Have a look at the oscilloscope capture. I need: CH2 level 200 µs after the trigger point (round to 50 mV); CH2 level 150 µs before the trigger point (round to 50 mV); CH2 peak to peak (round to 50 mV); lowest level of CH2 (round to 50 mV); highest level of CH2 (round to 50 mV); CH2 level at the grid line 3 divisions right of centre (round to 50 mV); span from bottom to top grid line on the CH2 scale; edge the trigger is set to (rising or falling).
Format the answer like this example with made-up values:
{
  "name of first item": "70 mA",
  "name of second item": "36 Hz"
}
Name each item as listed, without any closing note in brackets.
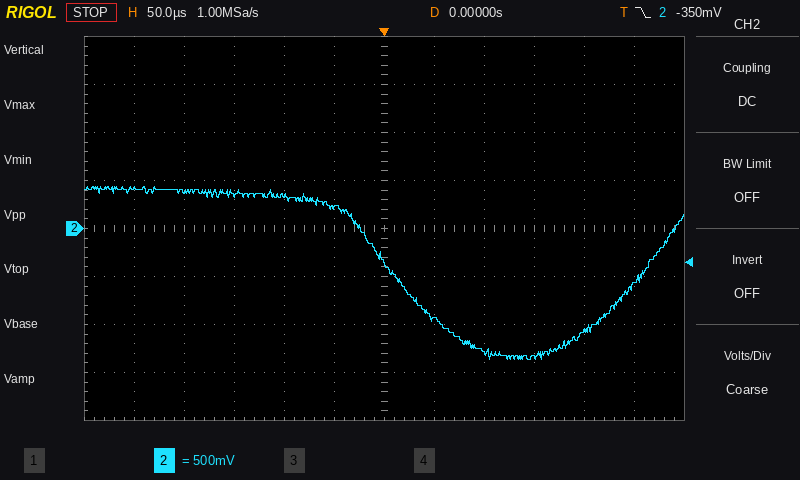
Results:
{
  "CH2 level 200 µs after the trigger point": "-1.05 V",
  "CH2 level 150 µs before the trigger point": "350 mV",
  "CH2 peak to peak": "1.80 V",
  "lowest level of CH2": "-1.35 V",
  "highest level of CH2": "450 mV",
  "CH2 level at the grid line 3 divisions right of centre": "-1.35 V",
  "span from bottom to top grid line on the CH2 scale": "4 V",
  "edge the trigger is set to": "falling"
}
